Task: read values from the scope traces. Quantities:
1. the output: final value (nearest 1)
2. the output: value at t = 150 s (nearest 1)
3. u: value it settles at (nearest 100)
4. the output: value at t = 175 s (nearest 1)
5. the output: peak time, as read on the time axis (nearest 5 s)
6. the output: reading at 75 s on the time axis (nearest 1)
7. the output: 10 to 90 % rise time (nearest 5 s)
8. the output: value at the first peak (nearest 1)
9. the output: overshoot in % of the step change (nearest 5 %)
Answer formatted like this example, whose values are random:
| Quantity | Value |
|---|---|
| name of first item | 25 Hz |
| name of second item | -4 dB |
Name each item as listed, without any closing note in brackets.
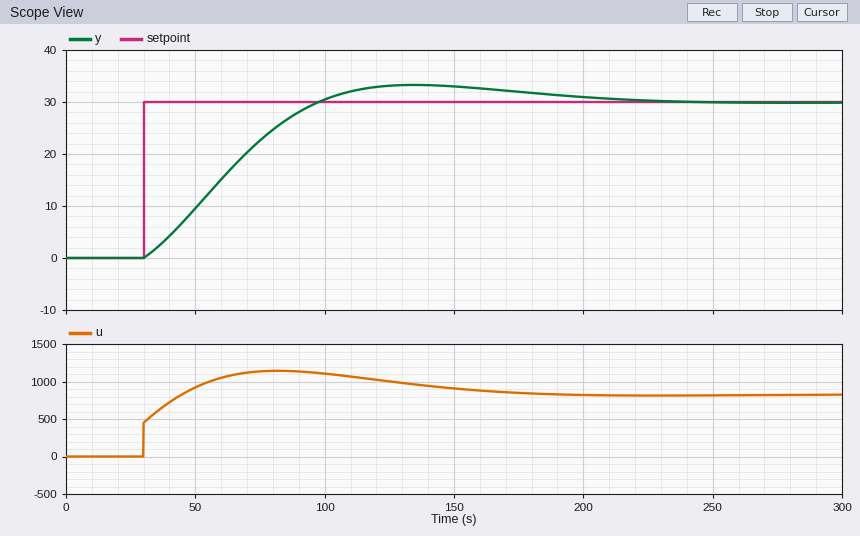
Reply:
| Quantity | Value |
|---|---|
| the output: final value | 30 |
| the output: value at t = 150 s | 33 |
| u: value it settles at | 800 |
| the output: value at t = 175 s | 32 |
| the output: peak time, as read on the time axis | 135 s |
| the output: reading at 75 s on the time axis | 23 |
| the output: 10 to 90 % rise time | 50 s |
| the output: value at the first peak | 33 |
| the output: overshoot in % of the step change | 10 % |
